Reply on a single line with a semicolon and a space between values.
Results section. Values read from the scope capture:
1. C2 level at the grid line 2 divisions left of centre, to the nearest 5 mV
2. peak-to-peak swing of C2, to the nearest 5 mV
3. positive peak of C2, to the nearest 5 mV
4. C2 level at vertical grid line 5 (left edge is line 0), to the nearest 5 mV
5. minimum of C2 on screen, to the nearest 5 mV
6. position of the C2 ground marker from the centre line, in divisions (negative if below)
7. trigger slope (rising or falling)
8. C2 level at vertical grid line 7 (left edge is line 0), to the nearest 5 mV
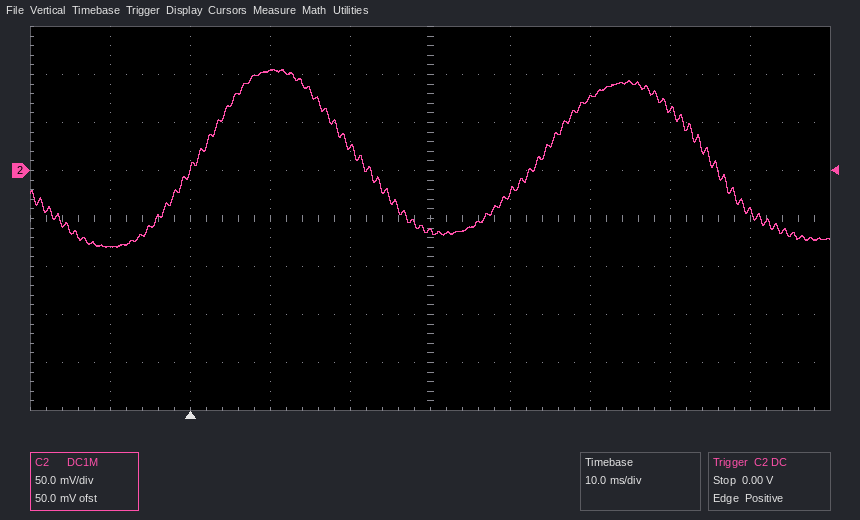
105 mV; 185 mV; 105 mV; -65 mV; -80 mV; +1.0 div; rising; 75 mV
